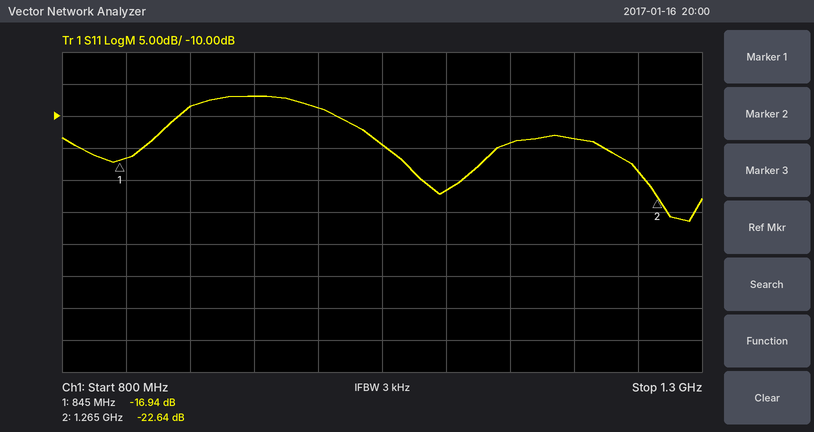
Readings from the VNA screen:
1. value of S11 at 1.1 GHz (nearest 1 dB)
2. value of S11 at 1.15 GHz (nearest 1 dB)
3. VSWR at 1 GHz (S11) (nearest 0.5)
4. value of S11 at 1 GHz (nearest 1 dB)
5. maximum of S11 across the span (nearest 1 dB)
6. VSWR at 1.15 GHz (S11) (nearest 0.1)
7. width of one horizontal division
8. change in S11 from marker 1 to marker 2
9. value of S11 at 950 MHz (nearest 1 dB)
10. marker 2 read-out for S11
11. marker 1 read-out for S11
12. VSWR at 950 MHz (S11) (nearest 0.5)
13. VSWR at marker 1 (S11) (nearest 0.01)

-22 dB
-14 dB
2.0
-9 dB
-7 dB
1.5
50 MHz
-5.70 dB
-7 dB
-22.64 dB
-16.94 dB
2.5
1.33
